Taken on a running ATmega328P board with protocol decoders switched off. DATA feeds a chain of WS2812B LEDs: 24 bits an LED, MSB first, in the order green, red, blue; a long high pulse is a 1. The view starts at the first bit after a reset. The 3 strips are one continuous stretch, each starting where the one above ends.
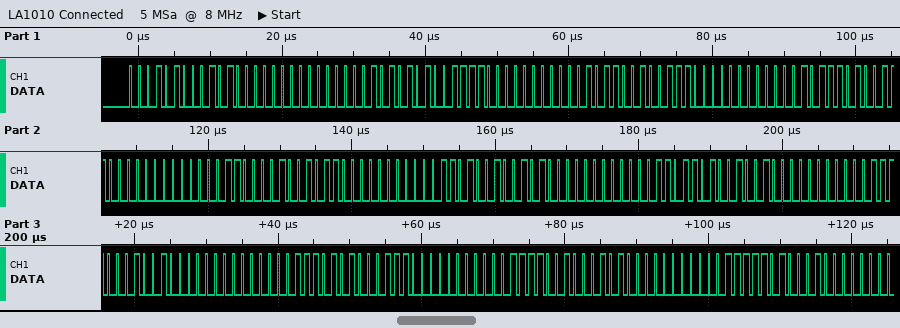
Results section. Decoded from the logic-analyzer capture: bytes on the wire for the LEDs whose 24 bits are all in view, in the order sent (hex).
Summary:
14 50 00 15 4F 00 16 4E 00 17 4C 00 18 4B 00 1A 4A 00 1B 49 00 1C 48 00 1D 47 00 1E 45 00
